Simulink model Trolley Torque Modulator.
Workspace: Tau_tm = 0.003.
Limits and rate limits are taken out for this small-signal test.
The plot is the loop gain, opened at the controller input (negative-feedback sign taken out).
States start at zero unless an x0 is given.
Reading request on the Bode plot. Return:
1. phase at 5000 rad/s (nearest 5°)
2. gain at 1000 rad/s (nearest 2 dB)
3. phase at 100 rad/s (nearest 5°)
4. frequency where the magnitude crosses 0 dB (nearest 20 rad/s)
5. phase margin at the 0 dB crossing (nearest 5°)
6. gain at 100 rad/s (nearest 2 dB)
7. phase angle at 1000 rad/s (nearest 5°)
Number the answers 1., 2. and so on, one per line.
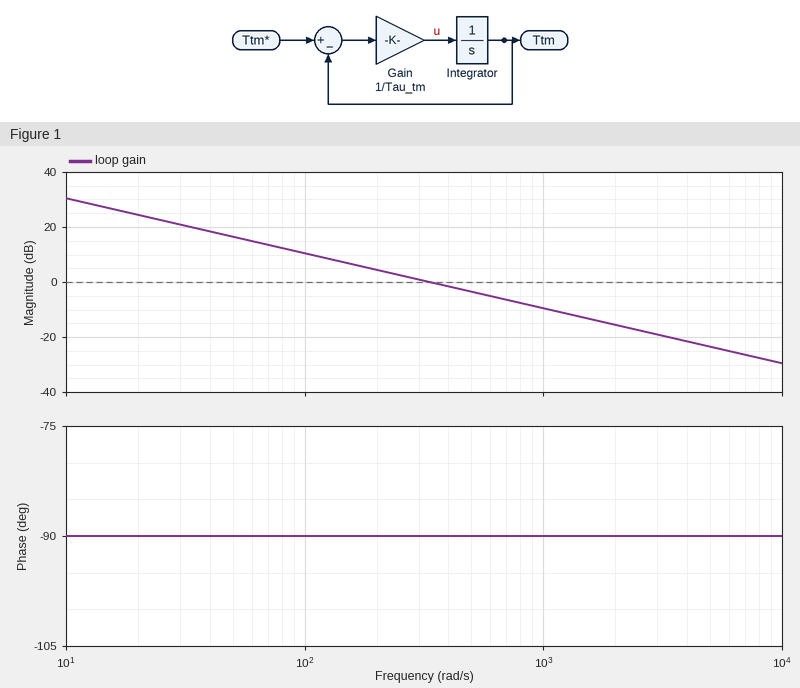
1. -90°
2. -10 dB
3. -90°
4. 340 rad/s
5. 90°
6. 10 dB
7. -90°
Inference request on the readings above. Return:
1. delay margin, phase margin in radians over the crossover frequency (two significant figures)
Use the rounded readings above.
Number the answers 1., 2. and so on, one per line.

1. 0.0046 s
